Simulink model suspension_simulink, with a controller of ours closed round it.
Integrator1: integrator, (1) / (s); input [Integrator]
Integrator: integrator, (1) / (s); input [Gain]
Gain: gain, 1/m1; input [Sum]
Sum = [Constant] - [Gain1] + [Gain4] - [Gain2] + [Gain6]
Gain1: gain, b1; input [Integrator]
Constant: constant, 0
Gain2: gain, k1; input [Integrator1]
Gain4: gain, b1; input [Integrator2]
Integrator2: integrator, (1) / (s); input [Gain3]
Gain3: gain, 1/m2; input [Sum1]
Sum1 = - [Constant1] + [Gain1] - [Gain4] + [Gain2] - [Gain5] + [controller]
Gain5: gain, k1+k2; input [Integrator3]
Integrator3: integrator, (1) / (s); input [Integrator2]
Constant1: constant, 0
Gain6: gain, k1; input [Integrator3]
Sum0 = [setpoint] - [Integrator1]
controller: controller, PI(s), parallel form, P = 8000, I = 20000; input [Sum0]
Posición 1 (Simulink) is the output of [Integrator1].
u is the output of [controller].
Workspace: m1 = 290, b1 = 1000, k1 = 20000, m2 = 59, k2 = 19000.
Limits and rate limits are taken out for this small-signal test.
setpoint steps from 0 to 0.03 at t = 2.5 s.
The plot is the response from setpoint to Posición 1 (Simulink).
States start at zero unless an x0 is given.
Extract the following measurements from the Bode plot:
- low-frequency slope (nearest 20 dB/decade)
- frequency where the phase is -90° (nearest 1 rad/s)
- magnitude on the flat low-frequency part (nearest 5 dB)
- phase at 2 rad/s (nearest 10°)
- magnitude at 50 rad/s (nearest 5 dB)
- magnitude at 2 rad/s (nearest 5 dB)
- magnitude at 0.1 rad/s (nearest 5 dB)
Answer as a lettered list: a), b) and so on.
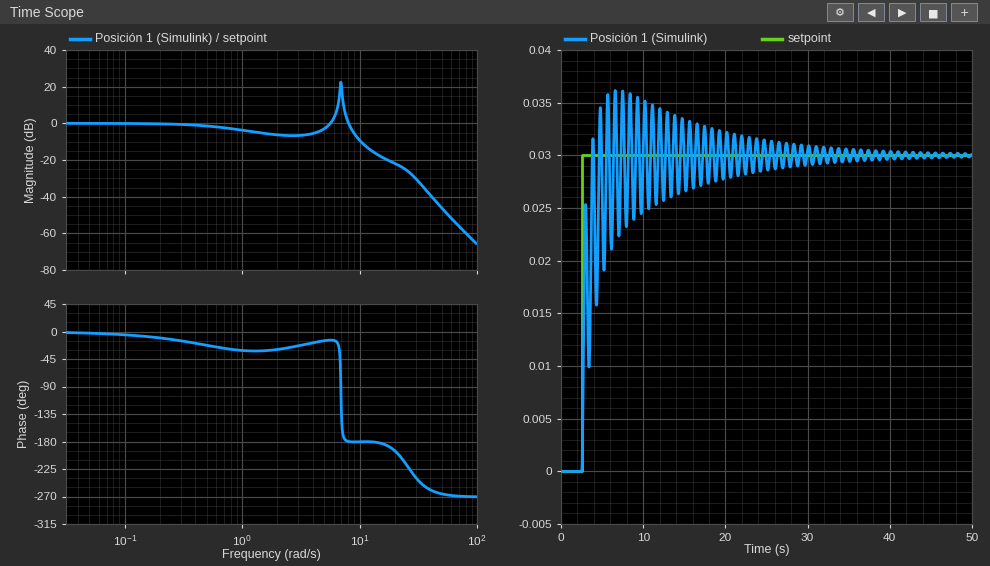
a) 0 dB/decade
b) 7 rad/s
c) 0 dB
d) -30°
e) -45 dB
f) -5 dB
g) 0 dB
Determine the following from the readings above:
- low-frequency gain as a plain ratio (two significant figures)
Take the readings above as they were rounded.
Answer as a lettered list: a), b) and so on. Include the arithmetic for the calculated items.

a) 10^(0 / 20) = 1.0
